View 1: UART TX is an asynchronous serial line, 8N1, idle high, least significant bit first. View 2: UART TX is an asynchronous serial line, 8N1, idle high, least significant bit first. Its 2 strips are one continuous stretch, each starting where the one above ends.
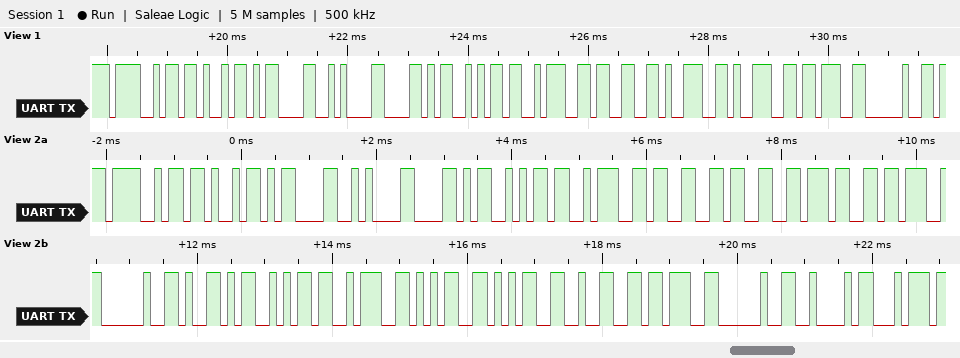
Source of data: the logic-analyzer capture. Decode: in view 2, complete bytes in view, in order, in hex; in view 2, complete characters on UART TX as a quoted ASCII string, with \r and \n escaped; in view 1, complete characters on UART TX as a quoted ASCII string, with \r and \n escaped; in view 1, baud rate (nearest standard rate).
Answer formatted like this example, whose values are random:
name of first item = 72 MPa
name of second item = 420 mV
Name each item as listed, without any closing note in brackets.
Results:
in view 2, complete bytes in view, in order, in hex = 0x4F 0x4B 0x0D 0x0A 0x58 0x6A 0x3A 0x33 0x33 0x37 0x3B 0x20 0x59 0x6A 0x3A 0x35 0x35 0x32 0x3B 0x20 0x42 0x74
in view 2, complete characters on UART TX as a quoted ASCII string, with \r and \n escaped = "OK\r\nXj:337; Yj:552; Bt"
in view 1, complete characters on UART TX as a quoted ASCII string, with \r and \n escaped = "OK\r\nXj:399; "
in view 1, baud rate = 9600 baud
